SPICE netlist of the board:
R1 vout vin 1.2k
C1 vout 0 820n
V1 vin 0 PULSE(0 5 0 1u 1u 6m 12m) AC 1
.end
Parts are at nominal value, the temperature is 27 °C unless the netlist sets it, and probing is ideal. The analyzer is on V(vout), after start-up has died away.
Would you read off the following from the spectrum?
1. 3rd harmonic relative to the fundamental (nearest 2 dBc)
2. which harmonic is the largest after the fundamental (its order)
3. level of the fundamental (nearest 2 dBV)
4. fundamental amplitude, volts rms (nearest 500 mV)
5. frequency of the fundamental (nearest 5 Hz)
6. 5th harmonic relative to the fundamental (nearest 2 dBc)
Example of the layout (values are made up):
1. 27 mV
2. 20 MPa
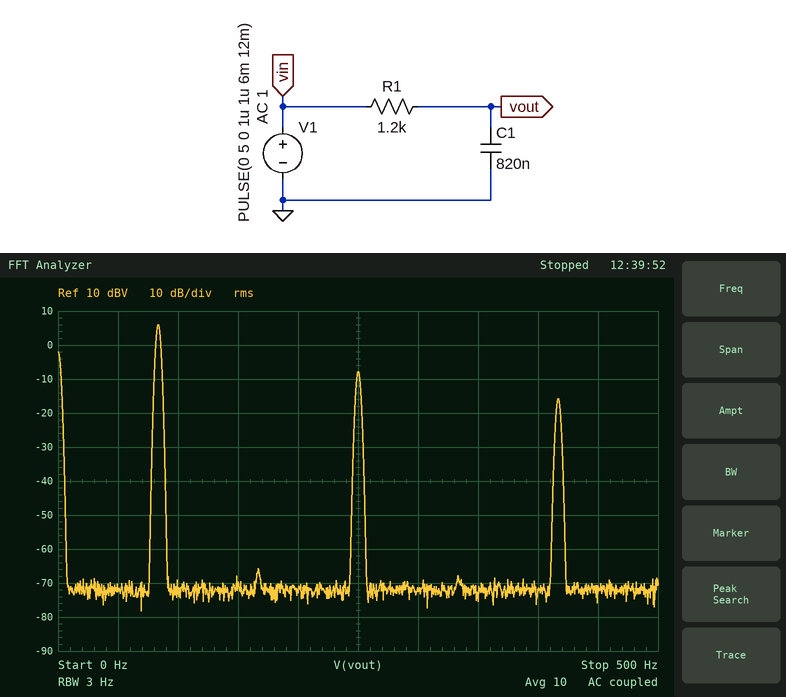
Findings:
1. -14 dBc
2. 3
3. 6 dBV
4. 2.0 V
5. 85 Hz
6. -22 dBc
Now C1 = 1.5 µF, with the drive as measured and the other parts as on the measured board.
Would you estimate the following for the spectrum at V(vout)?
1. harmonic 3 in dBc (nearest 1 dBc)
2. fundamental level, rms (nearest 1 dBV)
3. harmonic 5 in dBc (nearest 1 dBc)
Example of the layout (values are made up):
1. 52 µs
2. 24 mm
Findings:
1. -16 dBc
2. 4 dBV
3. -25 dBc
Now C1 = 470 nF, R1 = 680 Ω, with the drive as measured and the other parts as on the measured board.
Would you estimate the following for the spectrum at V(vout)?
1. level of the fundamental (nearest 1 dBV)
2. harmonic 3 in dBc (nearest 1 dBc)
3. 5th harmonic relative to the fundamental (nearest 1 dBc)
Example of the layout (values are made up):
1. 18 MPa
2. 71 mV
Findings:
1. 7 dBV
2. -10 dBc
3. -16 dBc
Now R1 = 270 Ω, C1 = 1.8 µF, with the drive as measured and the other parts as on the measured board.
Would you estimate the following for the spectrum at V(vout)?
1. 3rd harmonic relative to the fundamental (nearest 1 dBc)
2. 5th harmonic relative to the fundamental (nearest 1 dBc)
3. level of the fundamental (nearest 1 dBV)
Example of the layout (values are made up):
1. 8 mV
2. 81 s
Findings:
1. -11 dBc
2. -18 dBc
3. 7 dBV
